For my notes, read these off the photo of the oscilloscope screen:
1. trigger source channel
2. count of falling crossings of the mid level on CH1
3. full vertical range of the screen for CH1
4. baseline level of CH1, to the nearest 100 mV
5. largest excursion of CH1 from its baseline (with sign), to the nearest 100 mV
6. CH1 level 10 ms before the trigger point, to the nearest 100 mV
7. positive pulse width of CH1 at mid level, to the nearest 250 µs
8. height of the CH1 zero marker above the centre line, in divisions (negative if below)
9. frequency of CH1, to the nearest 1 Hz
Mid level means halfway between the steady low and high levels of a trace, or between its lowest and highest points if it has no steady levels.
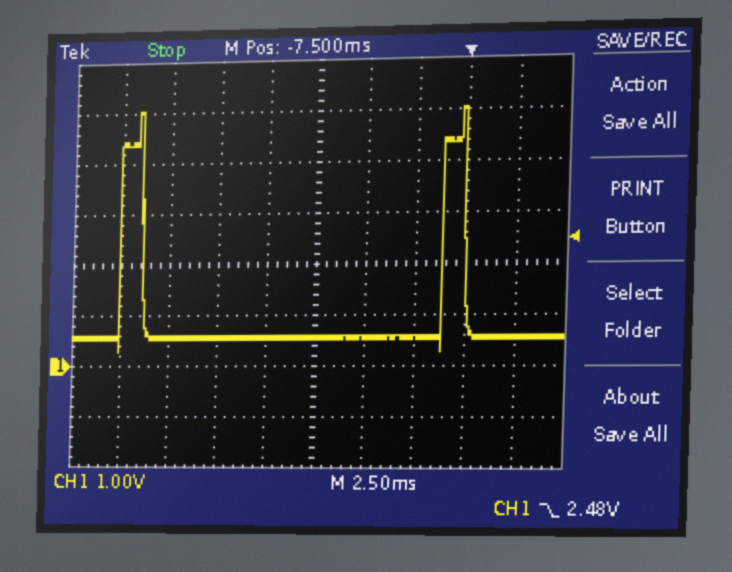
CH1
2
8 V
600 mV
+4.5 V
600 mV
1.25 ms
-2.0 div
61 Hz
